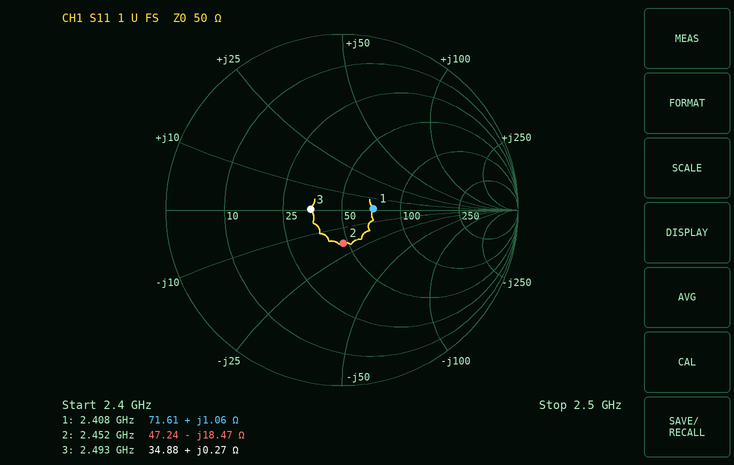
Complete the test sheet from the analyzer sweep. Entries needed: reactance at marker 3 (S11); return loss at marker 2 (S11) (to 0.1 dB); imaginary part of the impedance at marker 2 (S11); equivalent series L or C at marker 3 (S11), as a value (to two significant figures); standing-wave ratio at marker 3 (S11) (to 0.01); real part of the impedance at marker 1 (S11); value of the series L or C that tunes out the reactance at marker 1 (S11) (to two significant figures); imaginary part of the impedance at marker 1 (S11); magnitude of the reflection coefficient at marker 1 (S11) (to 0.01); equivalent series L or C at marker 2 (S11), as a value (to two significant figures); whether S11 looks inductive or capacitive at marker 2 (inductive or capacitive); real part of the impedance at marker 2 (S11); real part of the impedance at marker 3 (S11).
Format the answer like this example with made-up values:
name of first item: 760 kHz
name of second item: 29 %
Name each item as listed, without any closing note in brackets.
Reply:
reactance at marker 3: +0.27 Ω
return loss at marker 2 (S11): 14.5 dB
imaginary part of the impedance at marker 2: -18.47 Ω
equivalent series L or C at marker 3 (S11), as a value: 17 pH
standing-wave ratio at marker 3 (S11): 1.43
real part of the impedance at marker 1: 71.61 Ω
value of the series L or C that tunes out the reactance at marker 1 (S11): 62 pF
imaginary part of the impedance at marker 1: +1.06 Ω
magnitude of the reflection coefficient at marker 1 (S11): 0.18
equivalent series L or C at marker 2 (S11), as a value: 3.5 pF
whether S11 looks inductive or capacitive at marker 2: capacitive
real part of the impedance at marker 2: 47.24 Ω
real part of the impedance at marker 3: 34.88 Ω
